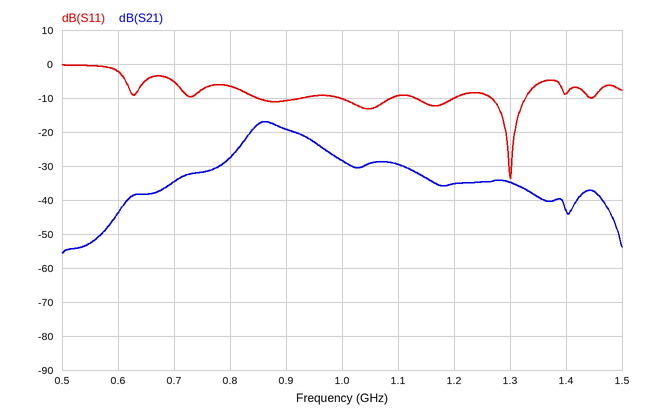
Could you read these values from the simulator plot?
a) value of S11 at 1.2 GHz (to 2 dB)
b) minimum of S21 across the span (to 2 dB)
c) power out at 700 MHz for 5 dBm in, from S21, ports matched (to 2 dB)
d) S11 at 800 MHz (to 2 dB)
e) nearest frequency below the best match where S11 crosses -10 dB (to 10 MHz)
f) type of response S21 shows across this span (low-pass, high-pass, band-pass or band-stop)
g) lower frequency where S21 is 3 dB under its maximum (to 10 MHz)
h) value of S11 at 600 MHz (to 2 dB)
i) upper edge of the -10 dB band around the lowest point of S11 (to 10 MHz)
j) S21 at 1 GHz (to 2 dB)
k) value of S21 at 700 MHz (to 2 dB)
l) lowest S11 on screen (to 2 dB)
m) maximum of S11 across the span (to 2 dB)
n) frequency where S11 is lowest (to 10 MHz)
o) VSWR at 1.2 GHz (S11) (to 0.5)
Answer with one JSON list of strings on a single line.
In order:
["-10 dB", "-56 dB", "-30 dBm", "-6 dB", "1.27 GHz", "band-pass", "840 MHz", "-2 dB", "1.33 GHz", "-28 dB", "-34 dB", "-34 dB", "0 dB", "1.30 GHz", "2.0"]
